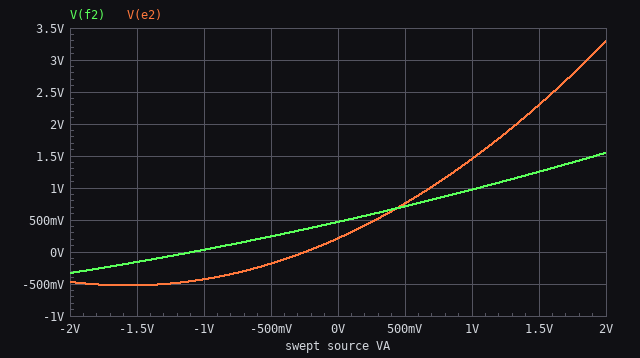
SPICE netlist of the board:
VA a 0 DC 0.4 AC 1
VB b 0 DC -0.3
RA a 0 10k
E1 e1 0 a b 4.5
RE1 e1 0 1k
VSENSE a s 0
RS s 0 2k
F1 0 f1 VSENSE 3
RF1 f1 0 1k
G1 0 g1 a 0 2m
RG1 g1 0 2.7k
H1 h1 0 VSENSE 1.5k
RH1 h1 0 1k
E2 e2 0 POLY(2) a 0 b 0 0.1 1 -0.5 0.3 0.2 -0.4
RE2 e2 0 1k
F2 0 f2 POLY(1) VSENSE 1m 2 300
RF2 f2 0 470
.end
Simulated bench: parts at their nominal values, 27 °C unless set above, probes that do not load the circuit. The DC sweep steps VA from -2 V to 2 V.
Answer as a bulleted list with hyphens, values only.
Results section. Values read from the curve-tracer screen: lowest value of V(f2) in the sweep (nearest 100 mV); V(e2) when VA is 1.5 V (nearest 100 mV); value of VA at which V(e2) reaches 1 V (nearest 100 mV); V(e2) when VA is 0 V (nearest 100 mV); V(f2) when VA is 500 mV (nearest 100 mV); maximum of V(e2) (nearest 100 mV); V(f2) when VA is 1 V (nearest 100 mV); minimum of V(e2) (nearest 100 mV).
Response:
- -300 mV
- 2.3 V
- 700 mV
- 200 mV
- 700 mV
- 3.3 V
- 1.0 V
- -500 mV
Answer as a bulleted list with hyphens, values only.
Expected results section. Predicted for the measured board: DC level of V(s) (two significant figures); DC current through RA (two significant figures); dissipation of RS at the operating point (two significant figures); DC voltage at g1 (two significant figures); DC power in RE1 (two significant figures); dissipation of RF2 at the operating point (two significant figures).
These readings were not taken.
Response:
- 400 mV
- 40 µA
- 80 µW
- 2.2 V
- 9.9 mW
- 940 µW
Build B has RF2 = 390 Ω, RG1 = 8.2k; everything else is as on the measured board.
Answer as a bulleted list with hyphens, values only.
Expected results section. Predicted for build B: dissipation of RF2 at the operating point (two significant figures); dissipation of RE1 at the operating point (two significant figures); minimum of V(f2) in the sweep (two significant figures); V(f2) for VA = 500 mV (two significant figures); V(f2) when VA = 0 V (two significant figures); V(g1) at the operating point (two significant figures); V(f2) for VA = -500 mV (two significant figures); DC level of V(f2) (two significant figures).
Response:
- 780 µW
- 9.9 mW
- -270 mV
- 590 mV
- 390 mV
- 6.6 V
- 200 mV
- 550 mV
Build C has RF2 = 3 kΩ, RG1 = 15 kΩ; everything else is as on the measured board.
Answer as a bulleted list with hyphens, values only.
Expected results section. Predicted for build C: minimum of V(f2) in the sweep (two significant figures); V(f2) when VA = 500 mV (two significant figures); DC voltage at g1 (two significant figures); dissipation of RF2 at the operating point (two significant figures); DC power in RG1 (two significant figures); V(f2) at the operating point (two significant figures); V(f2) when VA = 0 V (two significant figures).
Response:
- -2.1 V
- 4.6 V
- 12 V
- 6.0 mW
- 9.6 mW
- 4.2 V
- 3.0 V
